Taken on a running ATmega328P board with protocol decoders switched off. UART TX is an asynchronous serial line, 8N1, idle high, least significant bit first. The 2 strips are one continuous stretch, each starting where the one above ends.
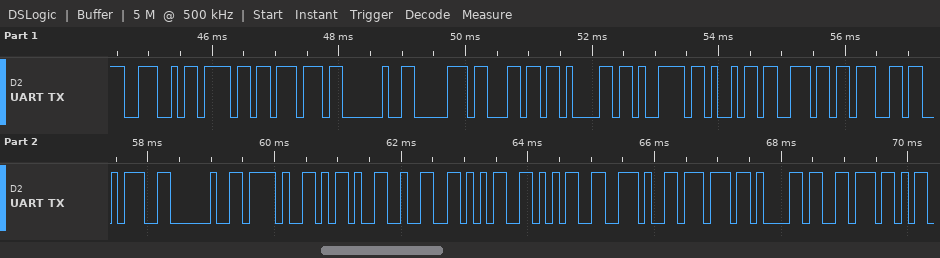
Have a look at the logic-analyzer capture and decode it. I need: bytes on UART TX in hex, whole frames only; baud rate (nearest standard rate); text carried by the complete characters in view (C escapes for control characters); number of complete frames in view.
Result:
4E 6F 77 20 70 6C 61 79 69 6E 67 3A 20 2F 2D 32 35 35 2E 77 61 76
9600 baud
"Now playing: /-255.wav"
22
